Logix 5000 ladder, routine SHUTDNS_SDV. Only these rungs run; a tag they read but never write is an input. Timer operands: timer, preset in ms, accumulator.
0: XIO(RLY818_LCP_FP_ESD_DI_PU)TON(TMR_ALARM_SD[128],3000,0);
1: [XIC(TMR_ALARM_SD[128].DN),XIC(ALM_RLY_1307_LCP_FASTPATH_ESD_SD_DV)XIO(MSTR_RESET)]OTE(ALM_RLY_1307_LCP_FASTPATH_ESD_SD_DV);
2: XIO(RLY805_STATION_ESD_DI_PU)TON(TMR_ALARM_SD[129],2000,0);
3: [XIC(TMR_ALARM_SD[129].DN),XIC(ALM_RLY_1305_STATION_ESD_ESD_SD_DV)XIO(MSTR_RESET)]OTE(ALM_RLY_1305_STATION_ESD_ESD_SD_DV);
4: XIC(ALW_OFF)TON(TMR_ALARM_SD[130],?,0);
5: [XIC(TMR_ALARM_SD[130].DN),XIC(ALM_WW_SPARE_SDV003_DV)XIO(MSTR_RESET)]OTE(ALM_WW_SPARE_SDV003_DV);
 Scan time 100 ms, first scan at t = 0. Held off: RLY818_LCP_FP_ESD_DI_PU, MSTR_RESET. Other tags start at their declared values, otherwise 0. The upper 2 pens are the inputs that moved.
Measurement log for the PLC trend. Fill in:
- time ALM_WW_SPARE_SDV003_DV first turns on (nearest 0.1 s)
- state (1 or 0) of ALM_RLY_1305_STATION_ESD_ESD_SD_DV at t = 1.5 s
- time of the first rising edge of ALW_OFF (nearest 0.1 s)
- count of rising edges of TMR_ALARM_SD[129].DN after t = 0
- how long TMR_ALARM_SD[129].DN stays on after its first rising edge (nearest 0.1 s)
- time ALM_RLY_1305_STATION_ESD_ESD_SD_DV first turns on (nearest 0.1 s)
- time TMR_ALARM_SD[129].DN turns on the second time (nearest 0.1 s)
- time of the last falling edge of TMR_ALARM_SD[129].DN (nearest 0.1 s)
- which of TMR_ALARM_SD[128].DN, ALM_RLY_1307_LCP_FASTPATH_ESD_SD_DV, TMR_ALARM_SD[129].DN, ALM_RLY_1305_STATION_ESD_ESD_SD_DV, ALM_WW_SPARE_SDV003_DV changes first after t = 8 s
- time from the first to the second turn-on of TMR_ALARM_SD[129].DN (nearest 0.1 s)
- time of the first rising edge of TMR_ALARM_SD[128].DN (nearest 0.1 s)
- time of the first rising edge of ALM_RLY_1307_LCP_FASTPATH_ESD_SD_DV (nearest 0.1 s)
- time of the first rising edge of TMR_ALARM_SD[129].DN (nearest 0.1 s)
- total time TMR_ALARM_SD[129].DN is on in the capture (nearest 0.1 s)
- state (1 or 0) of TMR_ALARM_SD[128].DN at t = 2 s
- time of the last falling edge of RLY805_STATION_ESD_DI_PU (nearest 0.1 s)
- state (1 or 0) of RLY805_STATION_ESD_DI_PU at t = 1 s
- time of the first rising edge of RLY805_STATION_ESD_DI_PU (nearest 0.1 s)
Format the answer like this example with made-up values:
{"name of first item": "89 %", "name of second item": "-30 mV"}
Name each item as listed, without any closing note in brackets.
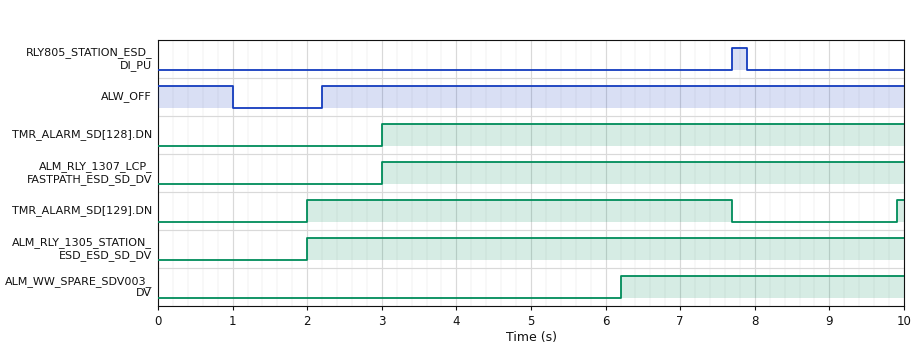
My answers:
{"time ALM_WW_SPARE_SDV003_DV first turns on": "6.2 s", "state (1 or 0) of ALM_RLY_1305_STATION_ESD_ESD_SD_DV at t = 1.5 s": "0", "time of the first rising edge of ALW_OFF": "2.2 s", "count of rising edges of TMR_ALARM_SD[129].DN after t = 0": "2", "how long TMR_ALARM_SD[129].DN stays on after its first rising edge": "5.7 s", "time ALM_RLY_1305_STATION_ESD_ESD_SD_DV first turns on": "2.0 s", "time TMR_ALARM_SD[129].DN turns on the second time": "9.9 s", "time of the last falling edge of TMR_ALARM_SD[129].DN": "7.7 s", "which of TMR_ALARM_SD[128].DN, ALM_RLY_1307_LCP_FASTPATH_ESD_SD_DV, TMR_ALARM_SD[129].DN, ALM_RLY_1305_STATION_ESD_ESD_SD_DV, ALM_WW_SPARE_SDV003_DV changes first after t = 8 s": "TMR_ALARM_SD[129].DN", "time from the first to the second turn-on of TMR_ALARM_SD[129].DN": "7.9 s", "time of the first rising edge of TMR_ALARM_SD[128].DN": "3.0 s", "time of the first rising edge of ALM_RLY_1307_LCP_FASTPATH_ESD_SD_DV": "3.0 s", "time of the first rising edge of TMR_ALARM_SD[129].DN": "2.0 s", "total time TMR_ALARM_SD[129].DN is on in the capture": "5.8 s", "state (1 or 0) of TMR_ALARM_SD[128].DN at t = 2 s": "0", "time of the last falling edge of RLY805_STATION_ESD_DI_PU": "7.9 s", "state (1 or 0) of RLY805_STATION_ESD_DI_PU at t = 1 s": "0", "time of the first rising edge of RLY805_STATION_ESD_DI_PU": "7.7 s"}
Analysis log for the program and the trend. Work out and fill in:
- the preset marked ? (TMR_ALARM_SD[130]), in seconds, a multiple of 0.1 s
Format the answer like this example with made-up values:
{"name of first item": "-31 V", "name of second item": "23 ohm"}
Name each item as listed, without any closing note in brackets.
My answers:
{"the preset marked ? (TMR_ALARM_SD[130]), in seconds, a multiple of 0.1 s": "4.0 s"}
